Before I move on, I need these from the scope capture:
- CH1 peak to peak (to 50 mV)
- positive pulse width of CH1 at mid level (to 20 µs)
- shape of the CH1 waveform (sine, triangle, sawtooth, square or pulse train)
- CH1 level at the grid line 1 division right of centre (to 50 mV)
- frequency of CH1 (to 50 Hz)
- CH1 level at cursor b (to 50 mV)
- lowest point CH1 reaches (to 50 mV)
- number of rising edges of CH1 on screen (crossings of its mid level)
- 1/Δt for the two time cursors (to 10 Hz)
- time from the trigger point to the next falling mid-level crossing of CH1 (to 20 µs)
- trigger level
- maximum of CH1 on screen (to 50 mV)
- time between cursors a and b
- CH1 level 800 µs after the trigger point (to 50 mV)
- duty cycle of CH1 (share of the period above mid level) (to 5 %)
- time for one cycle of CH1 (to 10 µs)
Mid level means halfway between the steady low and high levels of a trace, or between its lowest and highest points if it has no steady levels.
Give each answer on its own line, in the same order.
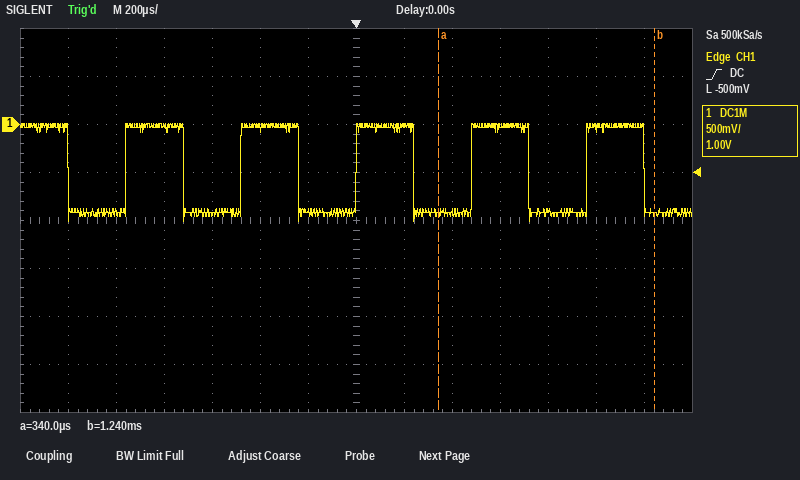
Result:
1.00 V
240 µs
square
0 mV
2.10 kHz
-950 mV
-1.00 V
5
1.11 kHz
240 µs
-500 mV
0 mV
900 µs
-900 mV
50 %
480 µs
